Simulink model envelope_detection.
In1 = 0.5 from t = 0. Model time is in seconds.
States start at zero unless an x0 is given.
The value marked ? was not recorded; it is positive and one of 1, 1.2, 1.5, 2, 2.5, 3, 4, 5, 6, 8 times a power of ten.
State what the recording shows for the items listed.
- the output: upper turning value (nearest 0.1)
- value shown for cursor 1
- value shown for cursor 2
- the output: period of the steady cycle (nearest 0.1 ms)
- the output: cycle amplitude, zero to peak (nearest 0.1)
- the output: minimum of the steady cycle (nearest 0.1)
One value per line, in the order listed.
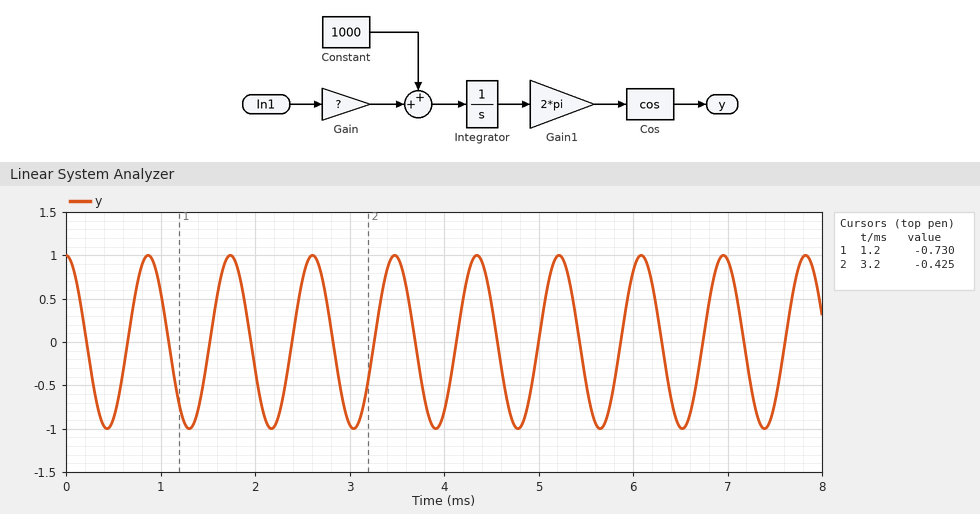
1.0
-0.730
-0.425
0.9 ms
1.0
-1.0
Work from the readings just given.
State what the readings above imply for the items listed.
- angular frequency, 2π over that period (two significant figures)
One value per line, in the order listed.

7.0 rad/ms
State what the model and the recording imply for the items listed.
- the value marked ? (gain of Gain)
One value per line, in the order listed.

300
